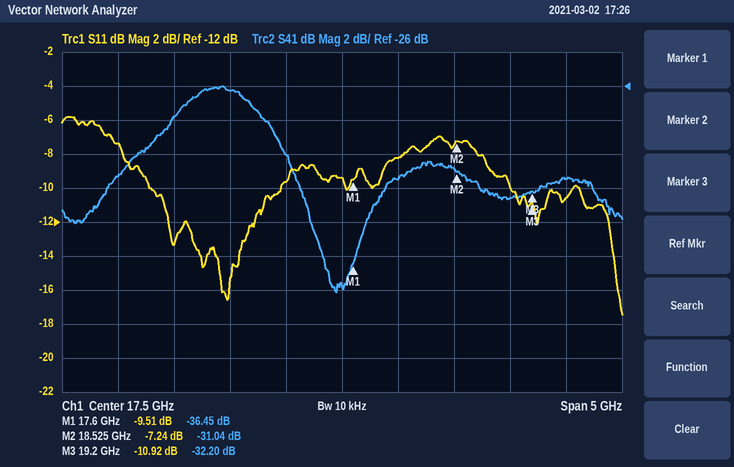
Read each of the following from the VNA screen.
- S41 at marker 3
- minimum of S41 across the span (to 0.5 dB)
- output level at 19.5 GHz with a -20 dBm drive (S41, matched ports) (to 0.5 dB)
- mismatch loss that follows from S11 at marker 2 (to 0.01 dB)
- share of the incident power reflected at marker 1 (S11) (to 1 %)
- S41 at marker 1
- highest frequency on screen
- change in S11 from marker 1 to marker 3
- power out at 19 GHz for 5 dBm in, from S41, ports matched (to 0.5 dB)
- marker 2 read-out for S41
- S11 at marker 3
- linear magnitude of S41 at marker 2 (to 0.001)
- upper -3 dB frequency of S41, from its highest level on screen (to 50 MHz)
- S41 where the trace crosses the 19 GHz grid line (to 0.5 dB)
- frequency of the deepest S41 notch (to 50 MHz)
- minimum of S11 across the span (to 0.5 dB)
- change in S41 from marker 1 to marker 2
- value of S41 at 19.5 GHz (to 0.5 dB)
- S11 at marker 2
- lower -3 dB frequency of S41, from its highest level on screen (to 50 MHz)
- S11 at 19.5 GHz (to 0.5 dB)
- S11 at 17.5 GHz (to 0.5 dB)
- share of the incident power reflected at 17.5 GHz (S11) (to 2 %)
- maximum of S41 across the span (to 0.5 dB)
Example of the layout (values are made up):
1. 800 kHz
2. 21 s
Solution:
1. -32.20 dB
2. -38.0 dB
3. -51.5 dBm
4. 0.91 dB
5. 11 %
6. -36.45 dB
7. 20 GHz
8. -1.41 dB
9. -27.5 dBm
10. -31.04 dB
11. -10.92 dB
12. 0.028
13. 16.90 GHz
14. -32.5 dB
15. 17.45 GHz
16. -17.5 dB
17. 5.41 dB
18. -31.5 dB
19. -7.24 dB
20. 15.85 GHz
21. -10.5 dB
22. -9.5 dB
23. 12 %
24. -26.0 dB
